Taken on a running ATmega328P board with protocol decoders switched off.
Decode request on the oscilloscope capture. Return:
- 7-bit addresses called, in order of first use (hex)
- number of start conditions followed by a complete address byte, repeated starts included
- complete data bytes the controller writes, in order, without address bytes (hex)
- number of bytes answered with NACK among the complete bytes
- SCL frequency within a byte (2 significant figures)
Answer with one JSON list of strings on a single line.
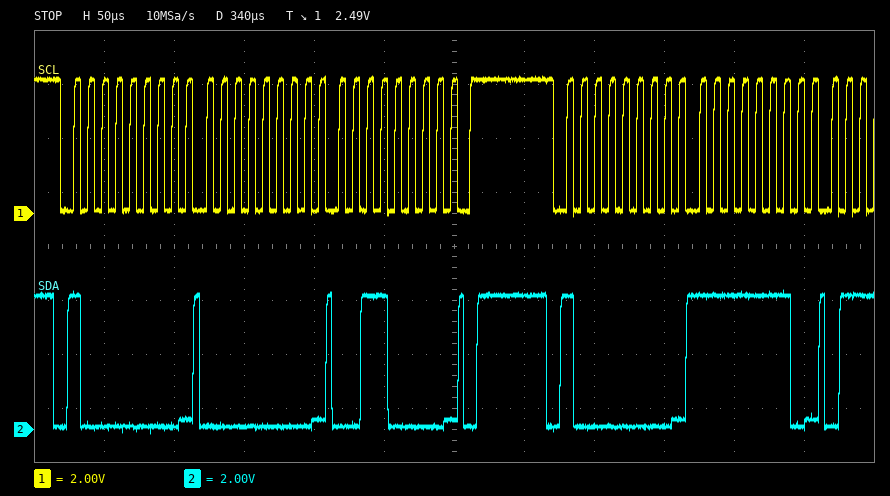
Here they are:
["0x40", "2", "00 30 FE", "0", "100 kHz"]
